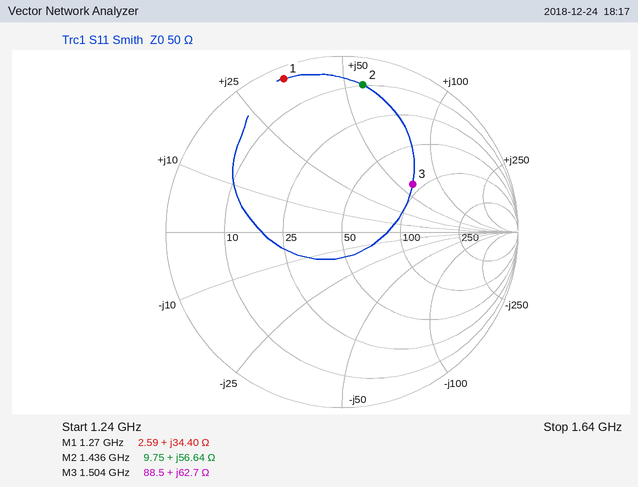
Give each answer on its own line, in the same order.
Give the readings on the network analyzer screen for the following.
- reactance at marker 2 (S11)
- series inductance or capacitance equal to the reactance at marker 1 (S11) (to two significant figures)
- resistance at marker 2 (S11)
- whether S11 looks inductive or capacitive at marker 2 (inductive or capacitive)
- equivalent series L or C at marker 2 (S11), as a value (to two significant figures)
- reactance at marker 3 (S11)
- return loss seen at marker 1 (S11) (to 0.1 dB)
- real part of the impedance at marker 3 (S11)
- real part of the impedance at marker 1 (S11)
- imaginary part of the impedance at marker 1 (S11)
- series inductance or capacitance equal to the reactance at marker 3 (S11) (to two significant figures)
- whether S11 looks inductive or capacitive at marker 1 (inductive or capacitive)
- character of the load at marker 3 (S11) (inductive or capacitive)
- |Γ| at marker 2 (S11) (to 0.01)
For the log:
+56.64 Ω
4.3 nH
9.75 Ω
inductive
6.3 nH
+62.7 Ω
0.6 dB
88.5 Ω
2.59 Ω
+34.40 Ω
6.6 nH
inductive
inductive
0.84
